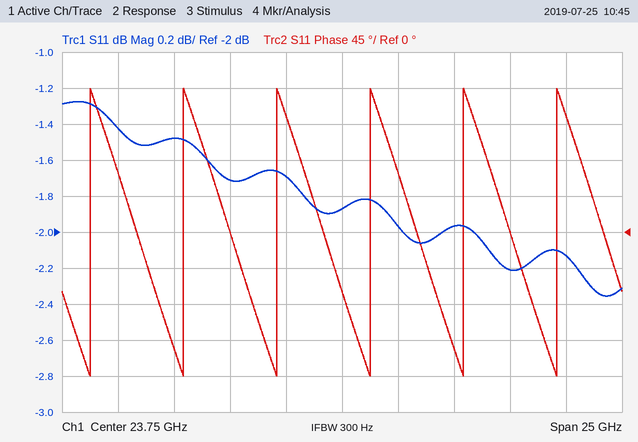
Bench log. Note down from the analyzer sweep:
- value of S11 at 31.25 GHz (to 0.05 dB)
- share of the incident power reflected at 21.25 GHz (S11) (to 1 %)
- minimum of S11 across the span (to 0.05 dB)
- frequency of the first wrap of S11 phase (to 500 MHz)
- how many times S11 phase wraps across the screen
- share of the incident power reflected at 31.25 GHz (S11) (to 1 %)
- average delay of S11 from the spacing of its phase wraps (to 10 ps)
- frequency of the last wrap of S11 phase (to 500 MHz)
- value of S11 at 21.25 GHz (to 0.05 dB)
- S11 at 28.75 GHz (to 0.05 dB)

-2.20 dB
68 %
-2.35 dB
12.5 GHz
6
60 %
240 ps
33.5 GHz
-1.70 dB
-1.95 dB
